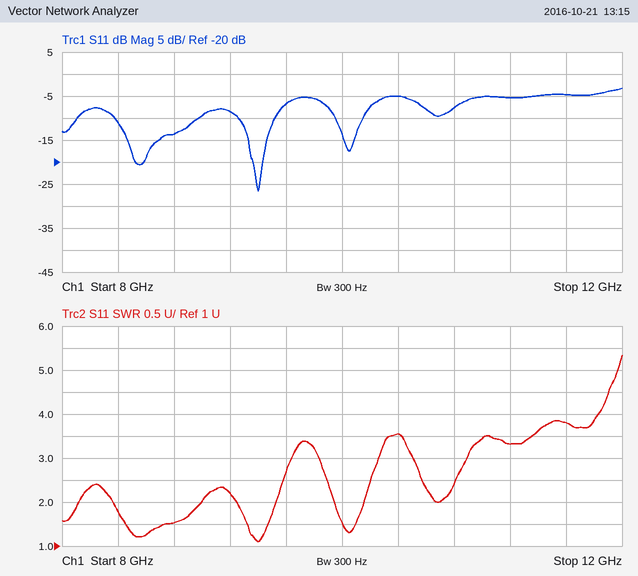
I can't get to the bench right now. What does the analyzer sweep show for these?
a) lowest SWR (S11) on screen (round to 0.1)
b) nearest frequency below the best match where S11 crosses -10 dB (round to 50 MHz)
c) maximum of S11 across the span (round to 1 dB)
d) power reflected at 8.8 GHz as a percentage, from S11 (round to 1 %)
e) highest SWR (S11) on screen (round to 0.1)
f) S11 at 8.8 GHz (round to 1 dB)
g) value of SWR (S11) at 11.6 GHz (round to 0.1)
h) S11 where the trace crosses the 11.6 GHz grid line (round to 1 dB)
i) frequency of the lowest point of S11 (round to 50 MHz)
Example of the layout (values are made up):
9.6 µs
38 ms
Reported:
1.1
9.25 GHz
-3 dB
4 %
5.3
-14 dB
3.8
-5 dB
9.40 GHz
